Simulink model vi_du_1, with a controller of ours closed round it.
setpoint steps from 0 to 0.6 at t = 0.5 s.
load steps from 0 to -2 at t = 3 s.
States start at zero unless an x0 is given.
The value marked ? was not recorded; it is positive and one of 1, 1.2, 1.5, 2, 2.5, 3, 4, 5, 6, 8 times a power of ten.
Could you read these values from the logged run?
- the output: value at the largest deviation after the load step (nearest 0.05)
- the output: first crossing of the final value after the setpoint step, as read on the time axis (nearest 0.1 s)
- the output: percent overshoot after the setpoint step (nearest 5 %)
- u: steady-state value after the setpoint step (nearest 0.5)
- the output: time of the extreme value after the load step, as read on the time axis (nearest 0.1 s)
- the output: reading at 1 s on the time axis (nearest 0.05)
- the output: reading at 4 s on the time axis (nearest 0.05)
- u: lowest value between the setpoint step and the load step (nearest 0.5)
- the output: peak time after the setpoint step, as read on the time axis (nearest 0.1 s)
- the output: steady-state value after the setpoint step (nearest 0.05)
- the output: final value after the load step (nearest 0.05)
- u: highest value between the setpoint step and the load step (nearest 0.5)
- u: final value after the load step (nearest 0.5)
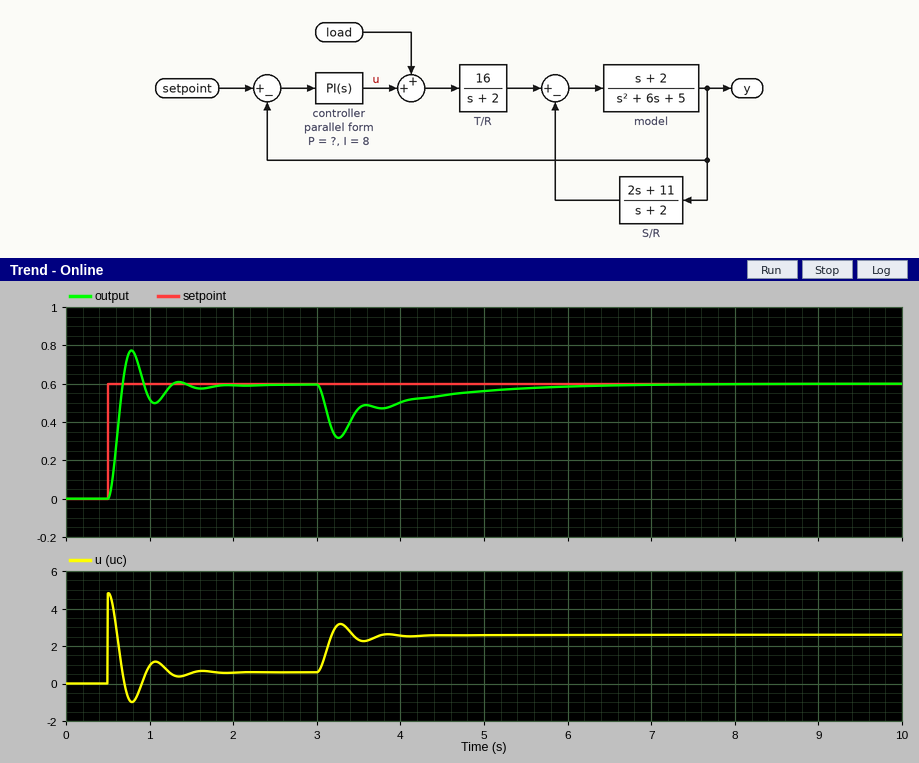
0.30
0.7 s
30 %
0.5
3.3 s
0.50
0.50
-1.0
0.8 s
0.60
0.60
5.0
2.5
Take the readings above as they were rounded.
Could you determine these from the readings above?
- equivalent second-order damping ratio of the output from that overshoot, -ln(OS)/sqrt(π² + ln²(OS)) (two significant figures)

0.36
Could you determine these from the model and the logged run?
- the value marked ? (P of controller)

8
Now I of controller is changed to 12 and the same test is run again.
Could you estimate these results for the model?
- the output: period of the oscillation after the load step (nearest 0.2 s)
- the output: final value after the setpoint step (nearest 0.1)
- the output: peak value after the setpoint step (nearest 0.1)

0.6 s
0.6
0.8
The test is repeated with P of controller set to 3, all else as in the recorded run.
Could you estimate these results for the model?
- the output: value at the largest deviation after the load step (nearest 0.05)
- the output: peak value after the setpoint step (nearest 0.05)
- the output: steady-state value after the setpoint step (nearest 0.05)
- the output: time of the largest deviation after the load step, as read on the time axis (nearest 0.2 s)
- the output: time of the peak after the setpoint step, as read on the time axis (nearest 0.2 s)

0.10
0.75
0.60
3.4 s
1.0 s
